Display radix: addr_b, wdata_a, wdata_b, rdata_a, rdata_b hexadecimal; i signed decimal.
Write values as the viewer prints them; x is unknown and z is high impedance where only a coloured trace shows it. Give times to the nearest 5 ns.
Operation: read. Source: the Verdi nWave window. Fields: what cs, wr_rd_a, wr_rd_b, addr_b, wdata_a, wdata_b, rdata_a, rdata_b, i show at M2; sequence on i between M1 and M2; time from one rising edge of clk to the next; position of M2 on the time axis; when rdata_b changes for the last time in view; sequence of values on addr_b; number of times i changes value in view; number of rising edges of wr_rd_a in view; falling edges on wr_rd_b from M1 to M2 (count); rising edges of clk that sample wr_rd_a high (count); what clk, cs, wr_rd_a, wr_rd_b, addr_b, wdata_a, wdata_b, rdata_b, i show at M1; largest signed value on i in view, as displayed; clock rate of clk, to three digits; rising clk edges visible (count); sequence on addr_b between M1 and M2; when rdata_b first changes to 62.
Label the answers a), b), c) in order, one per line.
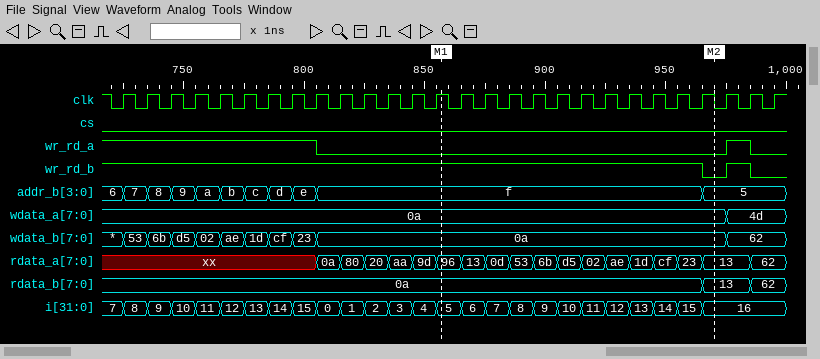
a) cs=0, wr_rd_a=0, wr_rd_b=0, addr_b=5, wdata_a=0a, wdata_b=0a, rdata_a=13, rdata_b=13, i=16
b) 5, 6, 7, 8, 9, 10, 11, 12, 13, 14, 15, 16
c) 10 ns
d) 970 ns
e) 985 ns
f) 6, 7, 8, 9, a, b, c, d, e, f, 5
g) 25
h) 1
i) 1
j) 10
k) clk=1, cs=0, wr_rd_a=0, wr_rd_b=1, addr_b=f, wdata_a=0a, wdata_b=0a, rdata_b=0a, i=5
l) 16
m) 100 MHz
n) 28
o) f, 5
p) 985 ns
